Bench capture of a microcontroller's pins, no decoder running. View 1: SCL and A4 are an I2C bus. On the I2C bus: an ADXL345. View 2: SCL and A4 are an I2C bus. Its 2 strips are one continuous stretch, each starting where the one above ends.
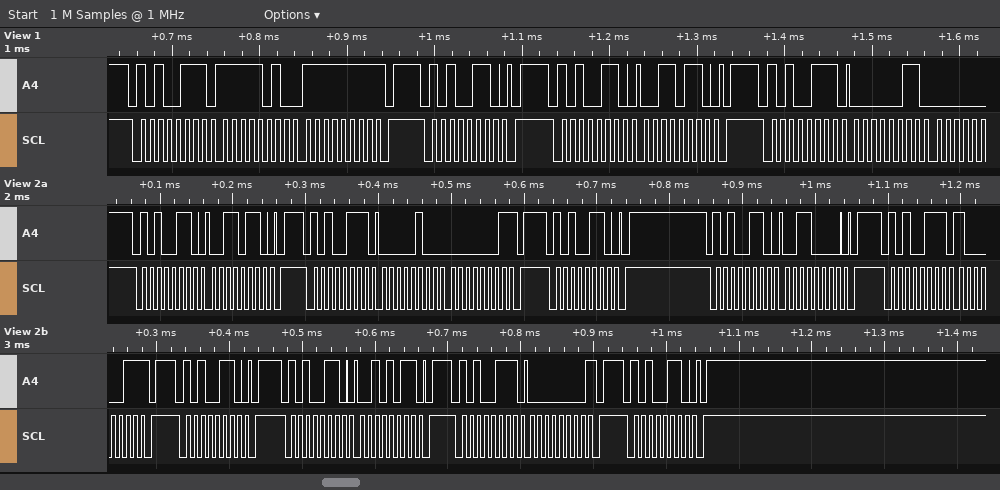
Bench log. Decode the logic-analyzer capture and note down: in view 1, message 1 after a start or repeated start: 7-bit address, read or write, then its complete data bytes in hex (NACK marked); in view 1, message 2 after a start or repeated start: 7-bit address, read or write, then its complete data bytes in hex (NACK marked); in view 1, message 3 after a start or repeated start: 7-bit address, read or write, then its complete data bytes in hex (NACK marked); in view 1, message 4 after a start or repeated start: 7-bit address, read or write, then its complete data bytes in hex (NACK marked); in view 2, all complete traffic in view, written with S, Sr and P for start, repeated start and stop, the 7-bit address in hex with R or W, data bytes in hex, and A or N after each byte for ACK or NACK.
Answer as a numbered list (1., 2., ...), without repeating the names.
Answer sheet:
1. 0x53 read: FA FF NACK
2. 0x53 write
3. 0x53 write: 36
4. 0x53 read: 03
5. S 53W A 36 A P S 53R A 04 A 01 N P S 53W A P S 53W A 30 A P S 53R A 83 N P S 53W A P S 53W A 2B A P S 53R A 00 N P S 53W A P
